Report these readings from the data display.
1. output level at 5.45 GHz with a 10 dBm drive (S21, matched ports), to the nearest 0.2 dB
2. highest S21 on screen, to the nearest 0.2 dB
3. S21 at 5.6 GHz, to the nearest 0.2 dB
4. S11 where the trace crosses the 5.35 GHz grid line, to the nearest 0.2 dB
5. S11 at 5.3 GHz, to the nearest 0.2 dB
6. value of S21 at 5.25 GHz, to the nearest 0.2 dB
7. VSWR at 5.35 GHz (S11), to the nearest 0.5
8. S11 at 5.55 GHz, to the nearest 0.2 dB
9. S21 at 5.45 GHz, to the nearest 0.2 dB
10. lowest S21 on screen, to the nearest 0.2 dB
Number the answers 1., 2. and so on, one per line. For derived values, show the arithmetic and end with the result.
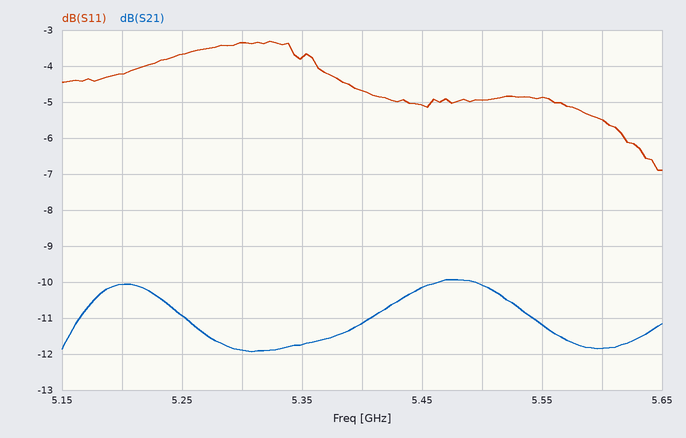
1. 10 dBm + (-10.2 dB) = -0.2 dBm
2. -10.0 dB
3. -11.8 dB
4. -3.8 dB
5. -3.4 dB
6. -11.0 dB
7. |Γ| = 10^(-3.8/20) = 0.6457; VSWR = (1 + 0.6457)/(1 − 0.6457) ≈ 4.64, so 4.5 to the nearest 0.5
8. -4.8 dB
9. -10.2 dB
10. -12.0 dB
